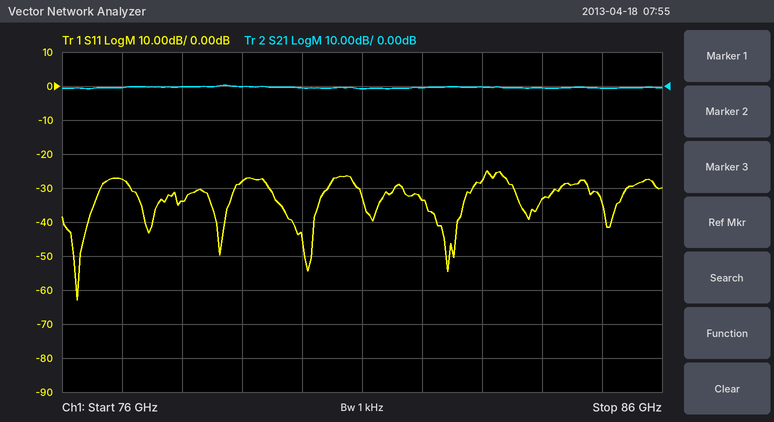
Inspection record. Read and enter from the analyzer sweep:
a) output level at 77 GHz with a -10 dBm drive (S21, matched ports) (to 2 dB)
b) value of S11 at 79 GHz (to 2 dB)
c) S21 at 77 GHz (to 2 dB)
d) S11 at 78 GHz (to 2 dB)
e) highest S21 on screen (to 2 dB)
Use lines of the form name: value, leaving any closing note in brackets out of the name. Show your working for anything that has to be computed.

output level at 77 GHz with a -10 dBm drive (S21, matched ports): -10 dBm + (0 dB) = -10 dBm
value of S11 at 79 GHz: -28 dB
S21 at 77 GHz: 0 dB
S11 at 78 GHz: -34 dB
highest S21 on screen: 0 dB
